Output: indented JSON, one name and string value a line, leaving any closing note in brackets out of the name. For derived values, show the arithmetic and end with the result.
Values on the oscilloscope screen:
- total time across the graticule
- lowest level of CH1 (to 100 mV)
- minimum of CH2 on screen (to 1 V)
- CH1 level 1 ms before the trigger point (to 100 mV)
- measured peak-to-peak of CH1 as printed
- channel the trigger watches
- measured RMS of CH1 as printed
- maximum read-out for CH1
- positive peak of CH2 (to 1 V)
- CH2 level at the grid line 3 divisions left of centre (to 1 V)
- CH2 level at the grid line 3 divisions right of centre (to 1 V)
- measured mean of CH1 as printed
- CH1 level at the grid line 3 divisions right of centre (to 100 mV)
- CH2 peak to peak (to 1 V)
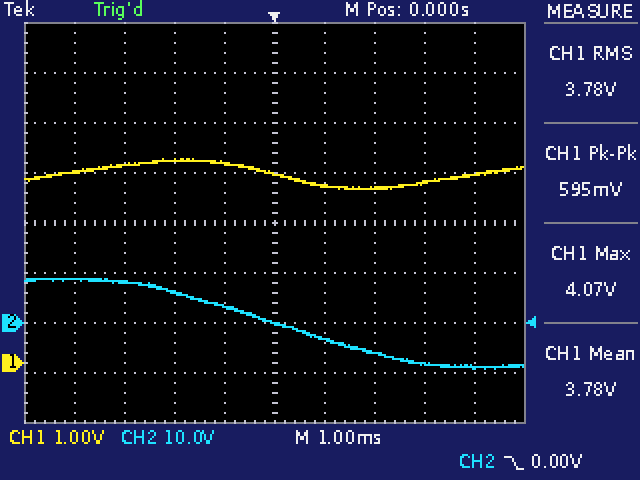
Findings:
{
  "total time across the graticule": "10 ms",
  "lowest level of CH1": "3.5 V",
  "minimum of CH2 on screen": "-9 V",
  "CH1 level 1 ms before the trigger point": "4.0 V",
  "measured peak-to-peak of CH1 as printed": "595 mV",
  "channel the trigger watches": "CH2",
  "measured RMS of CH1 as printed": "3.78 V",
  "maximum read-out for CH1": "4.07 V",
  "positive peak of CH2": "9 V",
  "CH2 level at the grid line 3 divisions left of centre": "8 V",
  "CH2 level at the grid line 3 divisions right of centre": "-8 V",
  "measured mean of CH1 as printed": "3.78 V",
  "CH1 level at the grid line 3 divisions right of centre": "3.6 V",
  "CH2 peak to peak": "9 V − (-9 V) = 18 V"
}
